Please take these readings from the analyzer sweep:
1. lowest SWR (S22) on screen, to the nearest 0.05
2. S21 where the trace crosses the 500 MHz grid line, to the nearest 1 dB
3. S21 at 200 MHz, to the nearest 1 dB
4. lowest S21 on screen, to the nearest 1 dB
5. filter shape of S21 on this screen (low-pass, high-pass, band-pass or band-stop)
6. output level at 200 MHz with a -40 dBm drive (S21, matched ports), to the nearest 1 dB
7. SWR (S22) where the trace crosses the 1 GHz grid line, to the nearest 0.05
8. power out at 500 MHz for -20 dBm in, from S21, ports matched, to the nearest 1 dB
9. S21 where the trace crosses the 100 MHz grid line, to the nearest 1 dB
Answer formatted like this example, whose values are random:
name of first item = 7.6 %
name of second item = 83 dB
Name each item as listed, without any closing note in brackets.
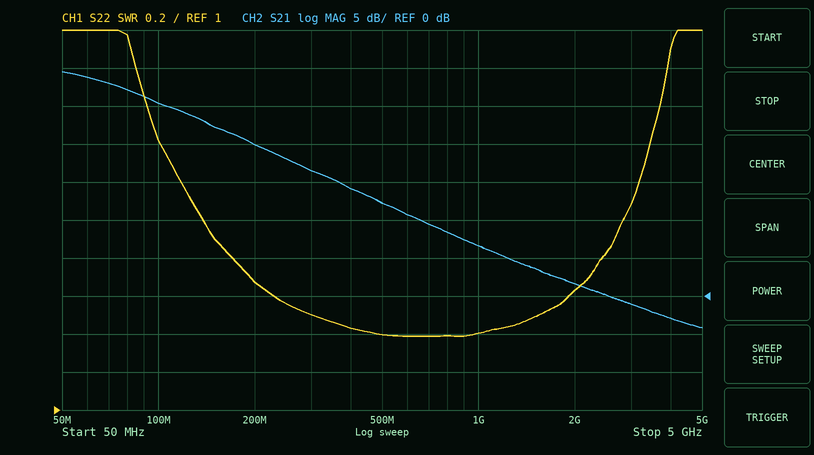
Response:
lowest SWR (S22) on screen, to the nearest 0.05 = 1.40
S21 where the trace crosses the 500 MHz grid line, to the nearest 1 dB = 12 dB
S21 at 200 MHz, to the nearest 1 dB = 20 dB
lowest S21 on screen, to the nearest 1 dB = -4 dB
filter shape of S21 on this screen = low-pass
output level at 200 MHz with a -40 dBm drive (S21, matched ports), to the nearest 1 dB = -20 dBm
SWR (S22) where the trace crosses the 1 GHz grid line, to the nearest 0.05 = 1.40
power out at 500 MHz for -20 dBm in, from S21, ports matched, to the nearest 1 dB = -8 dBm
S21 where the trace crosses the 100 MHz grid line, to the nearest 1 dB = 25 dB
